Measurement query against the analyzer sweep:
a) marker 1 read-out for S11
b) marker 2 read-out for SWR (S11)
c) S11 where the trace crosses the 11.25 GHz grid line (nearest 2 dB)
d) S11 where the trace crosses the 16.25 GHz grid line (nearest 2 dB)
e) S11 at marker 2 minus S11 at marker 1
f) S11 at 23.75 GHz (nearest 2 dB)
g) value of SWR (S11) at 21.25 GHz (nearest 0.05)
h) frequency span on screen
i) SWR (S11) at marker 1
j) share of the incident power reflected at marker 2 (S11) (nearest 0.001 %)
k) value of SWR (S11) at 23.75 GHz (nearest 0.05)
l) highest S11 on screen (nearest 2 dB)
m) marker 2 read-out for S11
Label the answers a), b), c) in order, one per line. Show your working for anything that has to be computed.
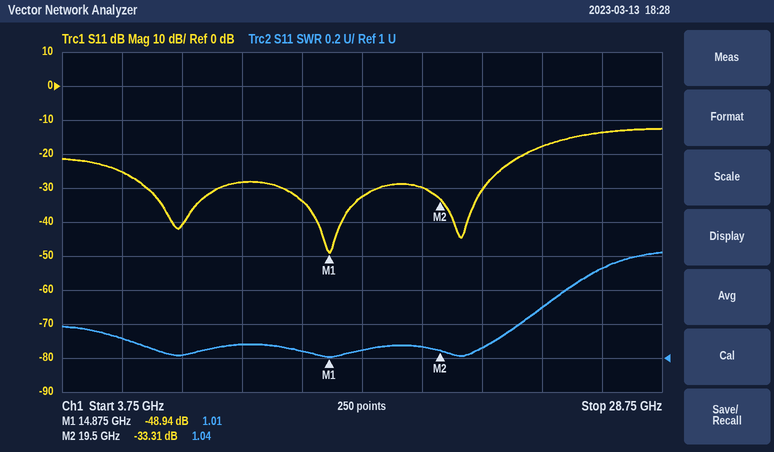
a) -48.94 dB
b) 1.04
c) -28 dB
d) -32 dB
e) -33.31 − (-48.94) = 15.63 dB
f) -18 dB
g) 1.05
h) 25 GHz
i) 1.01
j) 10^(-33.31/10) ≈ 0.047 %
k) 1.30
l) -12 dB
m) -33.31 dB
